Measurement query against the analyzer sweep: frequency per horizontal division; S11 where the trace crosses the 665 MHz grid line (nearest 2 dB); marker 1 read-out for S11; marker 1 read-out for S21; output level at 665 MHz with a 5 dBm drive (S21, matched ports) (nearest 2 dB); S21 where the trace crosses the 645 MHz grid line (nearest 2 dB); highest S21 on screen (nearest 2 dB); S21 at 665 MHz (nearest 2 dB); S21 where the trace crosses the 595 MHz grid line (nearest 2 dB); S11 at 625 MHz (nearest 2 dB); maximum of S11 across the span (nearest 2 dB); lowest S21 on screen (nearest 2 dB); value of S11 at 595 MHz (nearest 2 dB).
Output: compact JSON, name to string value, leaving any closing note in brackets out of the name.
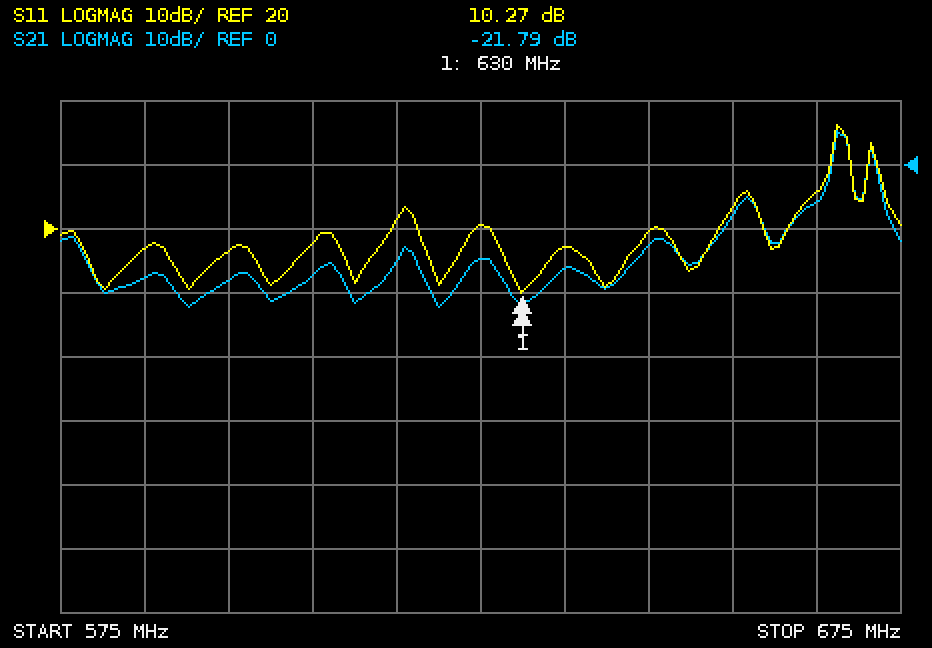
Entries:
{"frequency per horizontal division": "10 MHz", "S11 where the trace crosses the 665 MHz grid line": "26 dB", "marker 1 read-out for S11": "10.27 dB", "marker 1 read-out for S21": "-21.79 dB", "output level at 665 MHz with a 5 dBm drive (S21, matched ports)": "0 dBm", "S21 where the trace crosses the 645 MHz grid line": "-12 dB", "highest S21 on screen": "6 dB", "S21 at 665 MHz": "-6 dB", "S21 where the trace crosses the 595 MHz grid line": "-18 dB", "S11 at 625 MHz": "20 dB", "maximum of S11 across the span": "36 dB", "lowest S21 on screen": "-22 dB", "value of S11 at 595 MHz": "16 dB"}
